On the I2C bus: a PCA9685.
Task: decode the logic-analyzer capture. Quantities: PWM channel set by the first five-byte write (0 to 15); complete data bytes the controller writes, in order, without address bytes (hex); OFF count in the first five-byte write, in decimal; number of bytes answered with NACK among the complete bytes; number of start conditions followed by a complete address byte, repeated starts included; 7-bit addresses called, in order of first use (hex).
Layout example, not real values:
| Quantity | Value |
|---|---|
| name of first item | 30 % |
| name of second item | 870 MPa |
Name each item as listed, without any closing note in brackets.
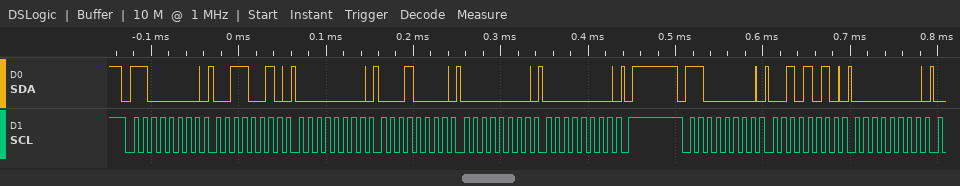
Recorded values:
| Quantity | Value |
|---|---|
| PWM channel set by the first five-byte write | 11 |
| complete data bytes the controller writes, in order, without address bytes | 32 00 10 00 00 2A 00 |
| OFF count in the first five-byte write, in decimal | 0 |
| number of bytes answered with NACK among the complete bytes | 0 |
| number of start conditions followed by a complete address byte, repeated starts included | 2 |
| 7-bit addresses called, in order of first use | 0x60 |
